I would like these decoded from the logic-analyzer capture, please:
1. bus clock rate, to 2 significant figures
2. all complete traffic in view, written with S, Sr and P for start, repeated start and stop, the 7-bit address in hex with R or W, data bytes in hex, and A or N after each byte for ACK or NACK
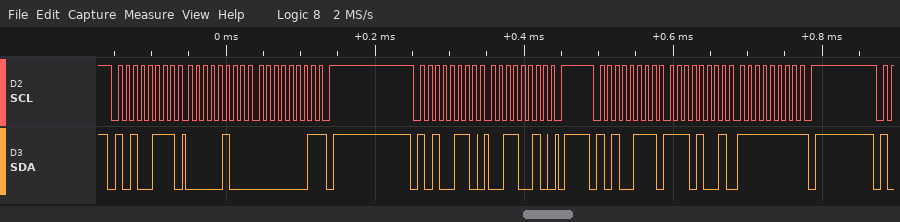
100 kHz
S 53R A 04 A 01 N P S 53W A 32 A P S 53R A E9 A FF N P
